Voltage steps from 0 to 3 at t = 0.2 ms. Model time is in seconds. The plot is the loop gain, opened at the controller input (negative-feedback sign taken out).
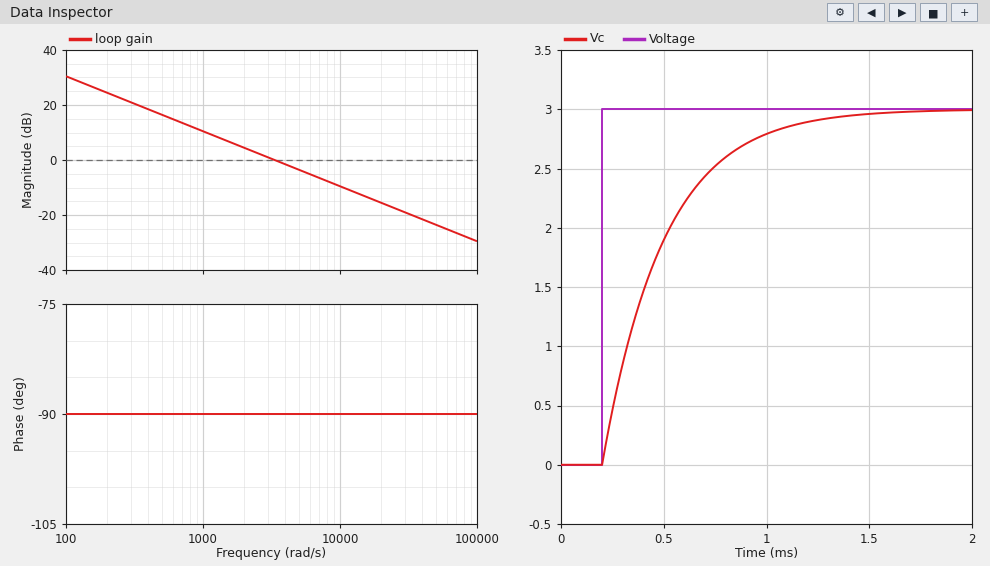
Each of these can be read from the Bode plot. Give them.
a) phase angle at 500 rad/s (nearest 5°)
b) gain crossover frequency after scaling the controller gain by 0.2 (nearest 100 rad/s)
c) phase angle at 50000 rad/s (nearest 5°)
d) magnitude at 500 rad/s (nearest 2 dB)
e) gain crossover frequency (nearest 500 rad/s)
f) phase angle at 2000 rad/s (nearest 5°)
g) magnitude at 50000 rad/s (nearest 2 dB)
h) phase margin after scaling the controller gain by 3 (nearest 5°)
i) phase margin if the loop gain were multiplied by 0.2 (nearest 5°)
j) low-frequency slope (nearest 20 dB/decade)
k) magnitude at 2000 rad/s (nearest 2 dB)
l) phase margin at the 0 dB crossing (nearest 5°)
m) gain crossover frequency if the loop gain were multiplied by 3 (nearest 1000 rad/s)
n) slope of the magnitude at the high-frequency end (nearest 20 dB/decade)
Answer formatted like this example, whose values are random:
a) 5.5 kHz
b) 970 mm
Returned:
a) -90°
b) 700 rad/s
c) -90°
d) 16 dB
e) 3500 rad/s
f) -90°
g) -24 dB
h) 90°
i) 90°
j) -20 dB/decade
k) 4 dB
l) 90°
m) 10000 rad/s
n) -20 dB/decade
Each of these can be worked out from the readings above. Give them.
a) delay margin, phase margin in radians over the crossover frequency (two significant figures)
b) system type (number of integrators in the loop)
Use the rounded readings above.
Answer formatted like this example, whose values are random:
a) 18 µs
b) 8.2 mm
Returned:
a) 0.00045 s
b) 1
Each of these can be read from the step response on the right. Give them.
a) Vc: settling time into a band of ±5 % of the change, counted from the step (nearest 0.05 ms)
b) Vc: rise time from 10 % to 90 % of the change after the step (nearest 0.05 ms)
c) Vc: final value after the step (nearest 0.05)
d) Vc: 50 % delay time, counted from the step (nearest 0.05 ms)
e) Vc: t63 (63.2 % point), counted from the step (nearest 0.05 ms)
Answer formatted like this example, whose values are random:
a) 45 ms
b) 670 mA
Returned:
a) 0.90 ms
b) 0.65 ms
c) 3.00
d) 0.20 ms
e) 0.30 ms
